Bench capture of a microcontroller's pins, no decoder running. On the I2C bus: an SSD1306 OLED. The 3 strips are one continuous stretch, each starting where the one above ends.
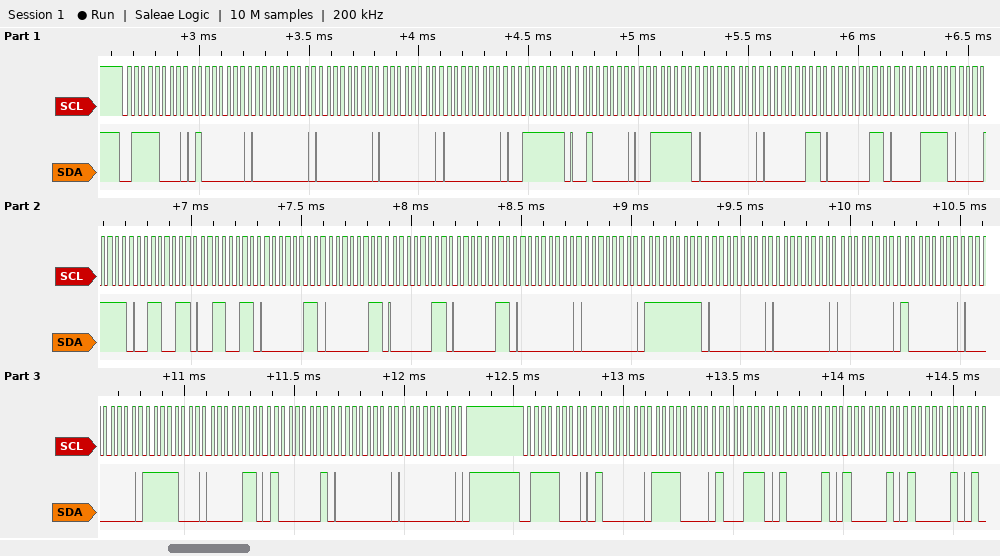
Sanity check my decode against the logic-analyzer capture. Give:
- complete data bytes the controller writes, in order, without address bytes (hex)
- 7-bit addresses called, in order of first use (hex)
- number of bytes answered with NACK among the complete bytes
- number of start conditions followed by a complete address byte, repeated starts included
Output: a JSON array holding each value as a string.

["40 00 00 00 00 3F 20 3F 00 03 03 0F 0F 33 33 03 03 03 03 00 00 FF 00 00 00 80 00 F8 06 81 00 00 40 F0 8E 82 82 82", "0x3C", "0", "2"]
